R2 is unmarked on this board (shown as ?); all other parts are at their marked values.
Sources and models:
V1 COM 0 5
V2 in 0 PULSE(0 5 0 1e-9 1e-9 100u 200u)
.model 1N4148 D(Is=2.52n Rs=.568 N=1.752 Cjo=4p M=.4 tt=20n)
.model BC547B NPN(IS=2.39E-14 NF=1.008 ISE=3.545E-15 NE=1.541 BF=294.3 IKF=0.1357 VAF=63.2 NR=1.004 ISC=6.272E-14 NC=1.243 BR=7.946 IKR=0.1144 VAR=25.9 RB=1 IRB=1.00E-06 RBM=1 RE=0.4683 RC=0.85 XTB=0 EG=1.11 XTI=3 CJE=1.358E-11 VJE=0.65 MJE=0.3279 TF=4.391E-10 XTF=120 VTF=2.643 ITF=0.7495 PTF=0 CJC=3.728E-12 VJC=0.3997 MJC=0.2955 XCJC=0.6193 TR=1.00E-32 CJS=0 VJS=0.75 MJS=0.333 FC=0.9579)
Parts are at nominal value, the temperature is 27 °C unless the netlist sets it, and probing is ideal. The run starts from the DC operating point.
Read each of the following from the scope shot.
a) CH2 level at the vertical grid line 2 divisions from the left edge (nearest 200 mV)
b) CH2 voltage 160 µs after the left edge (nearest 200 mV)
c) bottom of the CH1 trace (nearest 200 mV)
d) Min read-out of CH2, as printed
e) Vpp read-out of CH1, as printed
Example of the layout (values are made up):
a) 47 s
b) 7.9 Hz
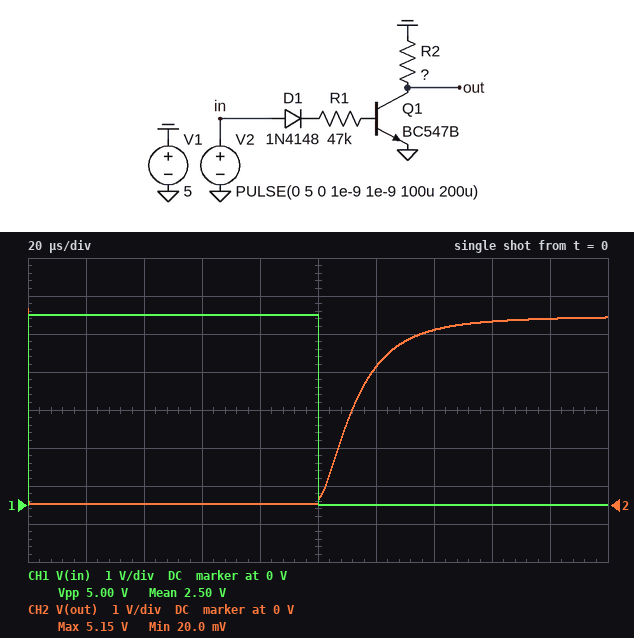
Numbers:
a) 0 V
b) 4.8 V
c) 0 V
d) 20.0 mV
e) 5.00 V
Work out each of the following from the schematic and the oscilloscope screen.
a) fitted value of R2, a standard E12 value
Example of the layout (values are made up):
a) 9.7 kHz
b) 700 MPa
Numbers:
a) 18 kΩ
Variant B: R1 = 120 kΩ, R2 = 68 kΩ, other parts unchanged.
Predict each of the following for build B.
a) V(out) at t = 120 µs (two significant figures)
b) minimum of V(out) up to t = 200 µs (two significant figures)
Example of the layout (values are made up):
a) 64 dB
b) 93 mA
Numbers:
a) 1.2 V
b) 12 mV
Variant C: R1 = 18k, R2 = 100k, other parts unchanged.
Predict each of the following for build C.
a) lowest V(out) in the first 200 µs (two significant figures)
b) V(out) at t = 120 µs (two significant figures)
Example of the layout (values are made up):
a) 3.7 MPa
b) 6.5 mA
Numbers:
a) 5.2 mV
b) 650 mV
